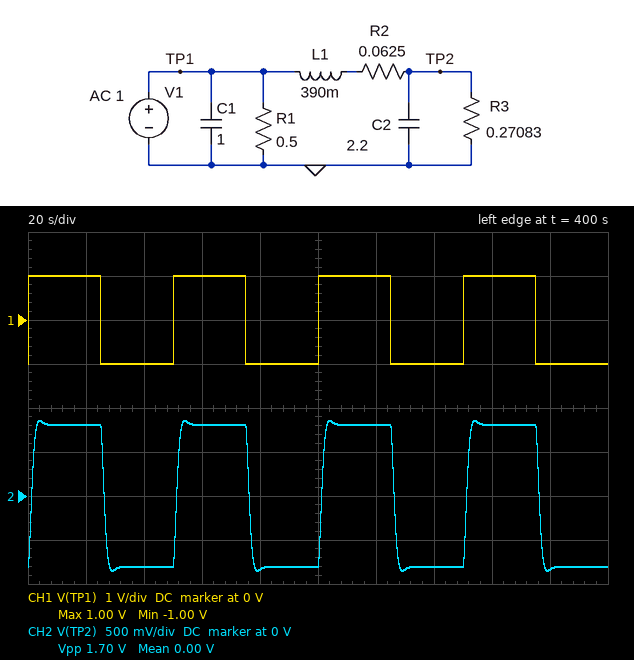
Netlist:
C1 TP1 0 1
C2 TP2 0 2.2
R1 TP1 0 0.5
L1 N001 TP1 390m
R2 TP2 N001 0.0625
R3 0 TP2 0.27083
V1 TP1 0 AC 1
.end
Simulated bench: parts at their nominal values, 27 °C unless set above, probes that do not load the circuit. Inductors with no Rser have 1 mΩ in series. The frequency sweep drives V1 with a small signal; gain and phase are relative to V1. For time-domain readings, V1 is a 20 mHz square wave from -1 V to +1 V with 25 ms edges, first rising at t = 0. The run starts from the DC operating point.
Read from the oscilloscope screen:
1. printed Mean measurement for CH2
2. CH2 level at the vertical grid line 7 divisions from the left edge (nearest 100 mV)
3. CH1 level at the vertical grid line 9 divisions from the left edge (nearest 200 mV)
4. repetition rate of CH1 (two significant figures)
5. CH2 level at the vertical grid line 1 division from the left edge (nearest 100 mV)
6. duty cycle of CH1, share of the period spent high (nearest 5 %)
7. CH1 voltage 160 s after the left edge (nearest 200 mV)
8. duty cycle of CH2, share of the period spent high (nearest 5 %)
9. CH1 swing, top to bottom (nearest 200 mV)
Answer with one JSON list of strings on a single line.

["0.00 V", "-800 mV", "-1.0 V", "20 mHz", "800 mV", "50 %", "1.0 V", "50 %", "2.0 V"]
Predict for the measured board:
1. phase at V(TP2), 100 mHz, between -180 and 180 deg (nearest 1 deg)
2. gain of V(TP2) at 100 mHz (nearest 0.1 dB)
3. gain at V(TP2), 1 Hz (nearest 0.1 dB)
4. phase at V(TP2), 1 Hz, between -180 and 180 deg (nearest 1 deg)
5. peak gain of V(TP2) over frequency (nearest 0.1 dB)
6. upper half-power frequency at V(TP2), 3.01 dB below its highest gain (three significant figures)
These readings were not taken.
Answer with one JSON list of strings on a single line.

["-48 deg", "-2.5 dB", "-30.7 dB", "-163 deg", "-1.8 dB", "175 mHz"]
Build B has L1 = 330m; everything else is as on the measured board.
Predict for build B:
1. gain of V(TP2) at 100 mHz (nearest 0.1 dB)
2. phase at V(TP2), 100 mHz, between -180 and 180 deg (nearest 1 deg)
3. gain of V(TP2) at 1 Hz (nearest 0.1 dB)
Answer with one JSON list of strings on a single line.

["-2.1 dB", "-42 deg", "-29.2 dB"]
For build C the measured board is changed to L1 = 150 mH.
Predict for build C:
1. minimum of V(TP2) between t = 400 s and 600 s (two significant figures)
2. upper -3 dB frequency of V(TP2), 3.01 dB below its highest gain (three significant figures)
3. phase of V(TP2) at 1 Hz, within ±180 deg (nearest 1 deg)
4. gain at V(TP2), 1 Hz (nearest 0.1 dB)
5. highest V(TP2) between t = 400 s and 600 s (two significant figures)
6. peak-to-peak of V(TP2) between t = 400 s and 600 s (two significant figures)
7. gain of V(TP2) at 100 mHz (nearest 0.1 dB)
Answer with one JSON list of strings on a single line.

["-1.0 V", "354 mHz", "-160 deg", "-22.0 dB", "1.0 V", "2.1 V", "-1.5 dB"]
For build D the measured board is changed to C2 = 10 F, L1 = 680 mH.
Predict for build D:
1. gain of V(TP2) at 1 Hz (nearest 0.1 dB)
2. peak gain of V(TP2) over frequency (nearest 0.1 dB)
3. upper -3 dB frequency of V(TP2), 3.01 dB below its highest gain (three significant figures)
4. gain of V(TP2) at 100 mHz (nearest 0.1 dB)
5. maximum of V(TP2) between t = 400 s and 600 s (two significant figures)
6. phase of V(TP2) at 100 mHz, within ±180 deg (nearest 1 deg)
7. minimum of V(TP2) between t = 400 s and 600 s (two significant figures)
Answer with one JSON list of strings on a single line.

["-48.6 dB", "-1.0 dB", "78.0 mHz", "-7.8 dB", "1.0 V", "-126 deg", "-1.0 V"]
